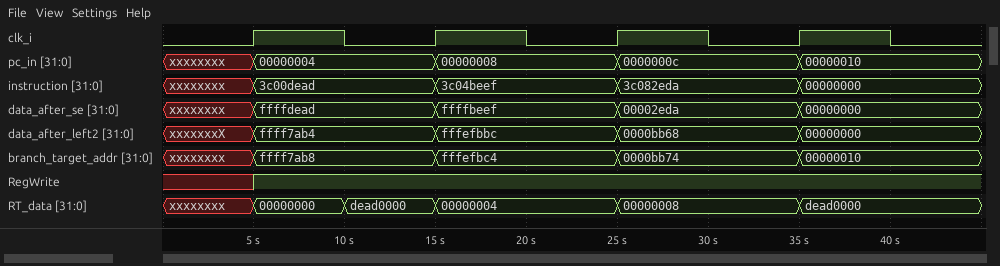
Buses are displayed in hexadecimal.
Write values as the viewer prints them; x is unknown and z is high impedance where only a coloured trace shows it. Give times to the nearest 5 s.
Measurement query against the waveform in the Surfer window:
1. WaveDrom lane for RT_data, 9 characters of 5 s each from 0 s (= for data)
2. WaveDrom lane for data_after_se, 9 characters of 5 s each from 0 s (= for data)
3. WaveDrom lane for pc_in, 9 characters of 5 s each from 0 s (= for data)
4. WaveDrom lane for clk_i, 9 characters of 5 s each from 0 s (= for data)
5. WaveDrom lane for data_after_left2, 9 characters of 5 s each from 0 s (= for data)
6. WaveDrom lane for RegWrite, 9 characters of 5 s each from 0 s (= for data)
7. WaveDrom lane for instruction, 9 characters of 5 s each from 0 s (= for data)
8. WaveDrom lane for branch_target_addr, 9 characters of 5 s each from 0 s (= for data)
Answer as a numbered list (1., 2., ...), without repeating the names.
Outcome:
1. {name: 'RT_data', wave: 'x===.=.=.', data: '00000000 dead0000 00000004 00000008 dead0000'}
2. {name: 'data_after_se', wave: 'x=.=.=.=.', data: 'ffffdead ffffbeef 00002eda 00000000'}
3. {name: 'pc_in', wave: 'x=.=.=.=.', data: '00000004 00000008 0000000c 00000010'}
4. {name: 'clk_i', wave: '010101010'}
5. {name: 'data_after_left2', wave: '==.=.=.=.', data: 'xxxxxxxX ffff7ab4 fffefbbc 0000bb68 00000000'}
6. {name: 'RegWrite', wave: 'x1.......'}
7. {name: 'instruction', wave: 'x=.=.=.=.', data: '3c00dead 3c04beef 3c082eda 00000000'}
8. {name: 'branch_target_addr', wave: 'x=.=.=.=.', data: 'ffff7ab8 fffefbc4 0000bb74 00000010'}
